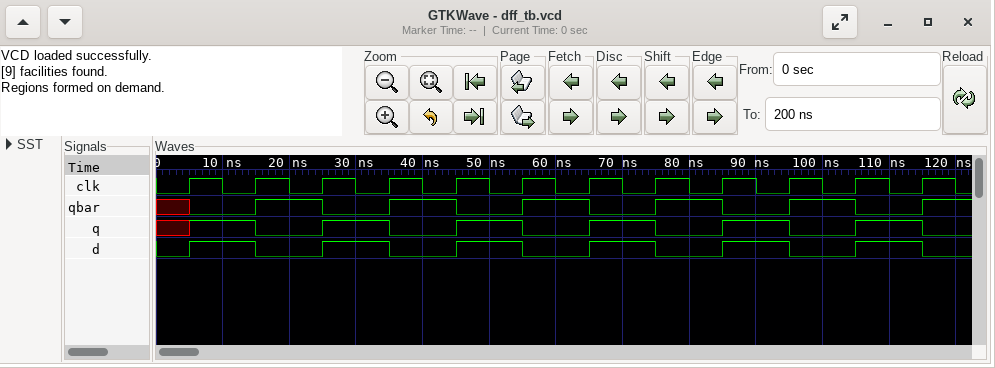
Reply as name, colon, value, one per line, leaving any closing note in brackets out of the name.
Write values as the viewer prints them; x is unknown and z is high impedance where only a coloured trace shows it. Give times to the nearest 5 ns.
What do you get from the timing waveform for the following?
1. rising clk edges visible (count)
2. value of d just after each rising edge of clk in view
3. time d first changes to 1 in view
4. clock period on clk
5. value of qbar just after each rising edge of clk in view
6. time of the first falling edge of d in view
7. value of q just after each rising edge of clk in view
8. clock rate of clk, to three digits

rising clk edges visible: 12
value of d just after each rising edge of clk in view: 1 0 1 0 1 0 1 0 1 0 1 0
time d first changes to 1 in view: 5 ns
clock period on clk: 10 ns
value of qbar just after each rising edge of clk in view: 0 1 0 1 0 1 0 1 0 1 0 1
time of the first falling edge of d in view: 15 ns
value of q just after each rising edge of clk in view: 1 0 1 0 1 0 1 0 1 0 1 0
clock rate of clk, to three digits: 100 MHz
